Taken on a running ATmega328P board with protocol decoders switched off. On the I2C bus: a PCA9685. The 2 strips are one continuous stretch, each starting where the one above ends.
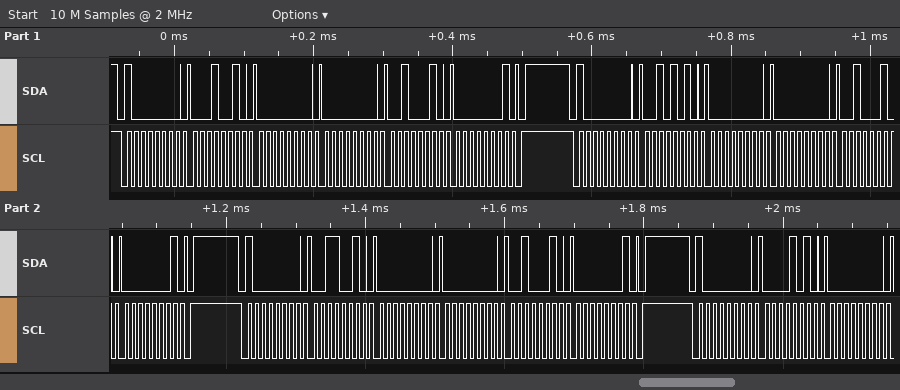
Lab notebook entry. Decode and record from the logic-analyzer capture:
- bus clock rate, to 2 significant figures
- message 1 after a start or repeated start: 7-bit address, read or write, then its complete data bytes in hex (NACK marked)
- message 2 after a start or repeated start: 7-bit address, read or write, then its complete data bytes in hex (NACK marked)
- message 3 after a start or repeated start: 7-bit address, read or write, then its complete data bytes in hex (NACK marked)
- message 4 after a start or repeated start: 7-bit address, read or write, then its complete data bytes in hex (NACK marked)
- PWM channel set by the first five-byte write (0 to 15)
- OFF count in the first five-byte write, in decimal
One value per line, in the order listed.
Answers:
100 kHz
0x40 write: 12 00 00 22 01
0x40 write: 2A 00 00 22 01
0x40 write: 32 00 00 22 01
0x40 write: 0A 00
3
290
